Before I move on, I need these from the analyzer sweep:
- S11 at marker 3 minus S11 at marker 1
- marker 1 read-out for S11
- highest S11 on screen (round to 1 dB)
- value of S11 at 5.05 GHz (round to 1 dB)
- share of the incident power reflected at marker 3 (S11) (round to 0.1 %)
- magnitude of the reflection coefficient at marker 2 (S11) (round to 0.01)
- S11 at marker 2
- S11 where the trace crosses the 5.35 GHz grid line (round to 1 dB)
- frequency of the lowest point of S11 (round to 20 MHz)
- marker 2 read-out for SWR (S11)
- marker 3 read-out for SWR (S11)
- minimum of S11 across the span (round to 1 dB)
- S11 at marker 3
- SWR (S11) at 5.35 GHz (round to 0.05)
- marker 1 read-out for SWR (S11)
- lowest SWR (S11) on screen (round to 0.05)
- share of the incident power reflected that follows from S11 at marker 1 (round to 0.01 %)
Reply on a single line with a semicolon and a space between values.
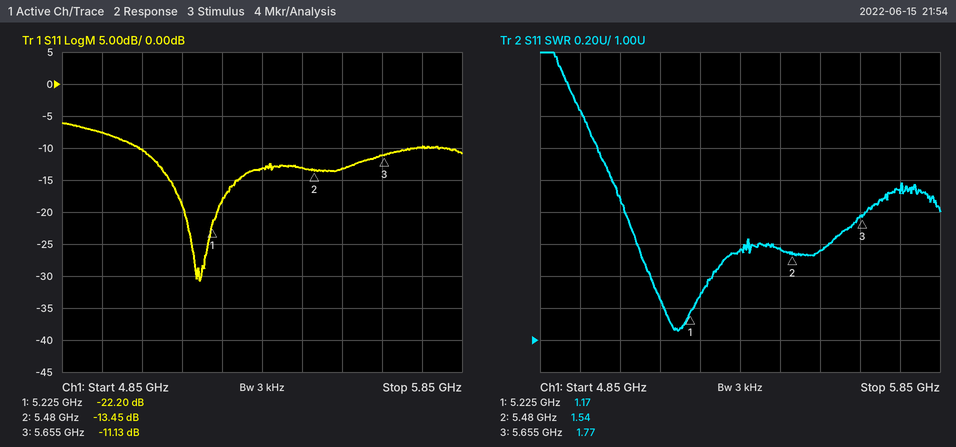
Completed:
11.07 dB; -22.20 dB; -6 dB; -10 dB; 7.7 %; 0.21; -13.45 dB; -13 dB; 5.20 GHz; 1.54; 1.77; -31 dB; -11.13 dB; 1.55; 1.17; 1.05; 0.60 %
